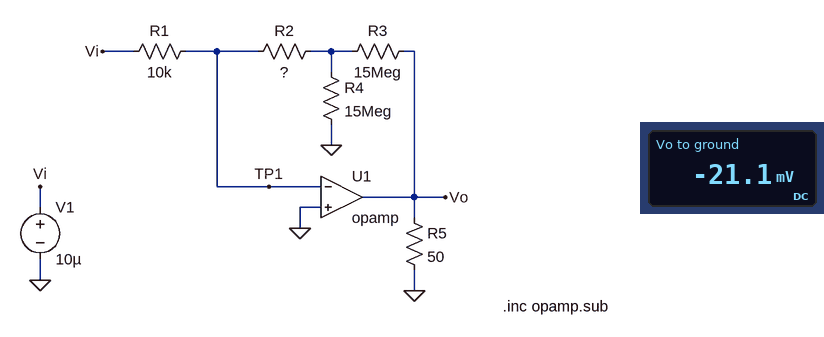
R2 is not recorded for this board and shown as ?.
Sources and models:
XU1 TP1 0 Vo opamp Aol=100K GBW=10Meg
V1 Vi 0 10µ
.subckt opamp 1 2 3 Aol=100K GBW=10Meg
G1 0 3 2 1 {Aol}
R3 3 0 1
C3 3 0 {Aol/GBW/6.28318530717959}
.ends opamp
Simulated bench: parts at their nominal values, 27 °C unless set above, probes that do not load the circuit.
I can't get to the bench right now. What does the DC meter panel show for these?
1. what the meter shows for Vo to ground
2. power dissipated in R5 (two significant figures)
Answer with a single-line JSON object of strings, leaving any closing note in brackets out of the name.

{"what the meter shows for Vo to ground": "-21.1 mV", "power dissipated in R5": "8.9 µW"}
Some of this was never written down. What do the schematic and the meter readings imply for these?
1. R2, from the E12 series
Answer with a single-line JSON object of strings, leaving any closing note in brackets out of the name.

{"R2, from the E12 series": "3.3 MΩ"}
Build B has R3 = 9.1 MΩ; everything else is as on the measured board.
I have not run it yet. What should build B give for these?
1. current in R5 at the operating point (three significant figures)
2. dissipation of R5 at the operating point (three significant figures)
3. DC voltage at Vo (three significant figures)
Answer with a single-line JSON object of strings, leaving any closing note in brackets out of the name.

{"current in R5 at the operating point": "284 µA", "dissipation of R5 at the operating point": "4.03 µW", "DC voltage at Vo": "-14.2 mV"}
